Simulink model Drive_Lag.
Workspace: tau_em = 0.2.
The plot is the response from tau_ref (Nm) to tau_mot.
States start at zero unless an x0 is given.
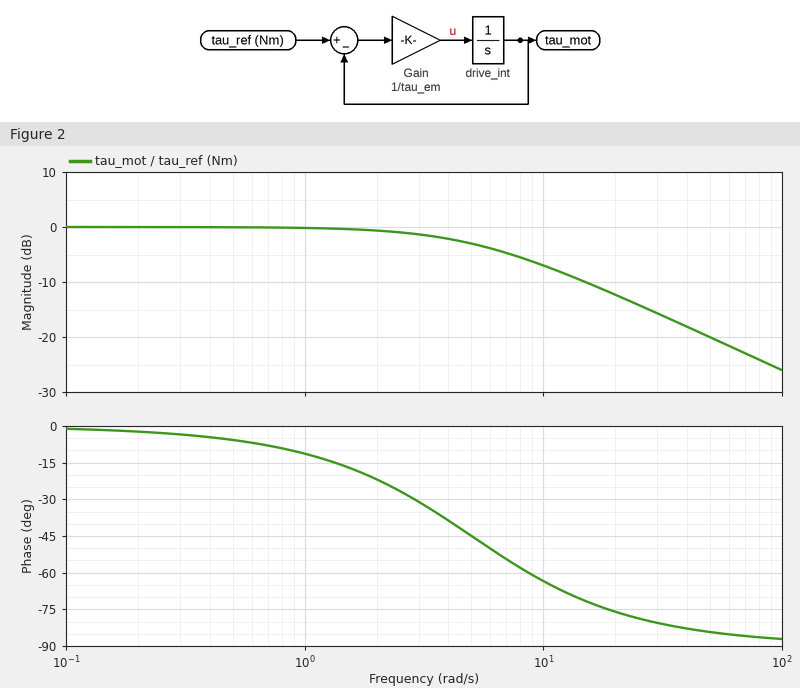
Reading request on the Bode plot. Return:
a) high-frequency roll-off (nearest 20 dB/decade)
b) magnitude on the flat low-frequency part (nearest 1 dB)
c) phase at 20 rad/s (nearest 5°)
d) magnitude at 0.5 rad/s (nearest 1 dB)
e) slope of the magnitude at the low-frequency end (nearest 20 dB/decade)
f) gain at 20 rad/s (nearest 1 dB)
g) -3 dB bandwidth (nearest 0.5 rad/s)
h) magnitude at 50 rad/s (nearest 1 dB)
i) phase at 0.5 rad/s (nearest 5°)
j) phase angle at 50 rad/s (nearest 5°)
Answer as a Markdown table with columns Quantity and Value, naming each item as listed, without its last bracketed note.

| Quantity | Value |
|---|---|
| high-frequency roll-off | -20 dB/decade |
| magnitude on the flat low-frequency part | 0 dB |
| phase at 20 rad/s | -75° |
| magnitude at 0.5 rad/s | 0 dB |
| slope of the magnitude at the low-frequency end | 0 dB/decade |
| gain at 20 rad/s | -12 dB |
| -3 dB bandwidth | 5.0 rad/s |
| magnitude at 50 rad/s | -20 dB |
| phase at 0.5 rad/s | -5° |
| phase angle at 50 rad/s | -85° |
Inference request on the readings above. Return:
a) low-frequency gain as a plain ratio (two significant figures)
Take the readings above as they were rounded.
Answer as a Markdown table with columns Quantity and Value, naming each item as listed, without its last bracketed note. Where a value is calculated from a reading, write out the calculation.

| Quantity | Value |
|---|---|
| low-frequency gain as a plain ratio | 10^(0 / 20) = 1.0 |
